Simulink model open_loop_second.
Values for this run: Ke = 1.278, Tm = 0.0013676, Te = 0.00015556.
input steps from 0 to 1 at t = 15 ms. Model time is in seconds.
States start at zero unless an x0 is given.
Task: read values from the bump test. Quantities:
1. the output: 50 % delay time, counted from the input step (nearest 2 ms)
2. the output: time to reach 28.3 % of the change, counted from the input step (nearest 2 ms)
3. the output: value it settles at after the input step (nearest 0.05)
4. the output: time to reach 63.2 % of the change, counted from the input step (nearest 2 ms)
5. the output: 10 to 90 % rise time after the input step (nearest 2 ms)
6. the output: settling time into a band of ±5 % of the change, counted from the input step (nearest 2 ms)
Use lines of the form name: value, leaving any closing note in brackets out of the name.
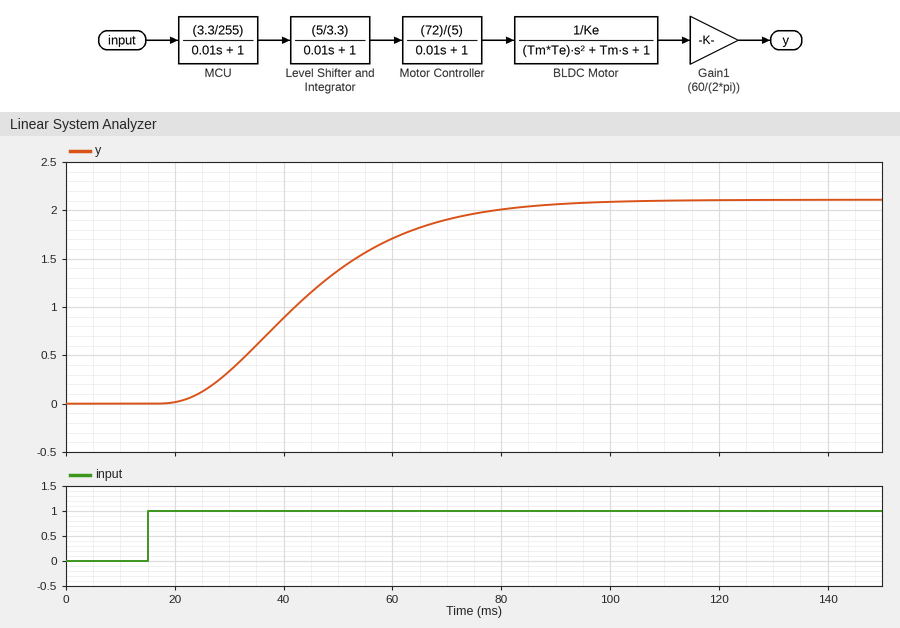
the output: 50 % delay time, counted from the input step: 28 ms
the output: time to reach 28.3 % of the change, counted from the input step: 20 ms
the output: value it settles at after the input step: 2.10
the output: time to reach 63.2 % of the change, counted from the input step: 34 ms
the output: 10 to 90 % rise time after the input step: 42 ms
the output: settling time into a band of ±5 % of the change, counted from the input step: 64 ms
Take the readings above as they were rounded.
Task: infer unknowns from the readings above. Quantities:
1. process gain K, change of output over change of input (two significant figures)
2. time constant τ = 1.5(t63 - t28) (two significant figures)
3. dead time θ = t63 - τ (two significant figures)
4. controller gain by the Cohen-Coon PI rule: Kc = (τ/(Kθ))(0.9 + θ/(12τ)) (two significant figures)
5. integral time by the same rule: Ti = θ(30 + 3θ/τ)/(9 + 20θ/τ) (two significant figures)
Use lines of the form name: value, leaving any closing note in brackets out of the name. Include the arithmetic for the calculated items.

process gain K, change of output over change of input: (2.1 - 0) / 1 = 2.1
time constant τ = 1.5(t63 - t28): 1.5 × (34 - 20) = 21 ms
dead time θ = t63 - τ: 34 - 21 = 13 ms
controller gain by the Cohen-Coon PI rule: Kc = (τ/(Kθ))(0.9 + θ/(12τ)): 21 / (2.1 × 13) × (0.9 + 13 / (12 × 21)) = 0.73
integral time by the same rule: Ti = θ(30 + 3θ/τ)/(9 + 20θ/τ): 13 × (30 + 3 × 13 / 21) / (9 + 20 × 13 / 21) = 19 ms
